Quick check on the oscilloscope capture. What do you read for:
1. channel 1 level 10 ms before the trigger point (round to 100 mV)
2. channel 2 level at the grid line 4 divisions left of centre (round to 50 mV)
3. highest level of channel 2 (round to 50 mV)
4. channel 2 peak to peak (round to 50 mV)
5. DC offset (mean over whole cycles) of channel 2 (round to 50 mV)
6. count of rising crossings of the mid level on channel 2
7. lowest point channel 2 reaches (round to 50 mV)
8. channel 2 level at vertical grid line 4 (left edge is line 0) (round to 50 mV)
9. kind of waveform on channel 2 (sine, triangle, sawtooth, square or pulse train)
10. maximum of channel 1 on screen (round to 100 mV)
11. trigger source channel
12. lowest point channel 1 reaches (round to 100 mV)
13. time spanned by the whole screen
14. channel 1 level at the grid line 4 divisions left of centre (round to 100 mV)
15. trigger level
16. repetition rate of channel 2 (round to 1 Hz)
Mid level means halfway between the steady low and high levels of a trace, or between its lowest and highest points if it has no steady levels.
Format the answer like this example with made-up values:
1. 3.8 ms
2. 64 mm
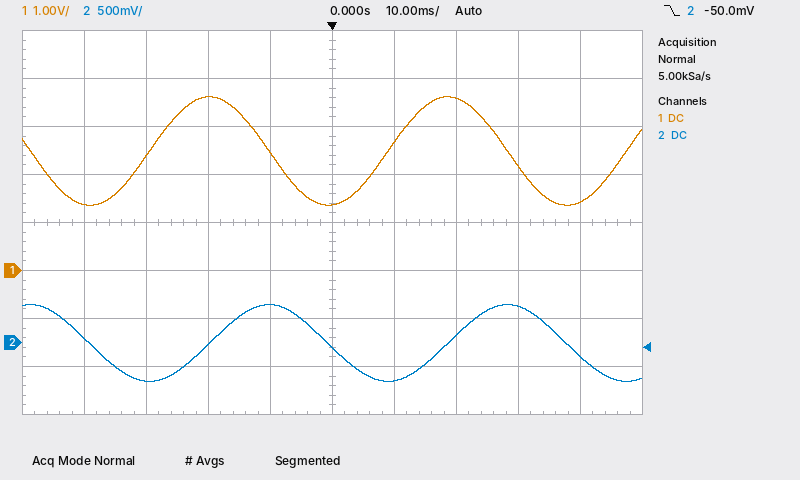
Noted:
1. 2.5 V
2. 50 mV
3. 400 mV
4. 800 mV
5. 0 mV
6. 2
7. -400 mV
8. 400 mV
9. sine
10. 3.6 V
11. channel 2
12. 1.4 V
13. 100 ms
14. 1.4 V
15. -50.0 mV
16. 26 Hz
